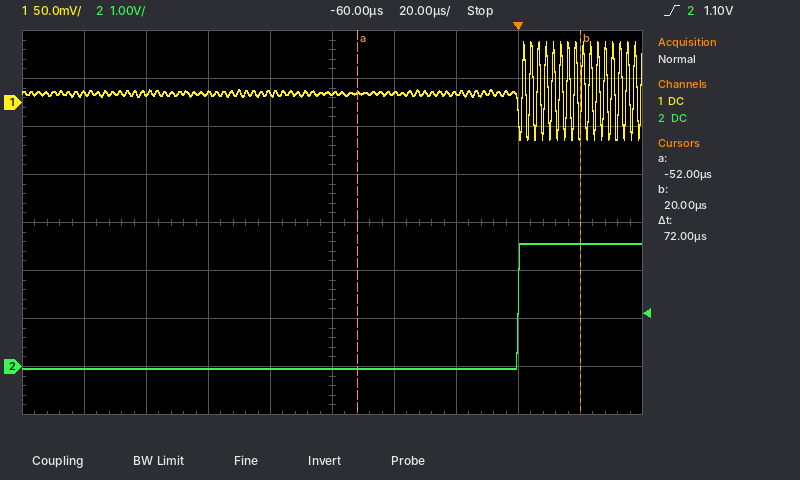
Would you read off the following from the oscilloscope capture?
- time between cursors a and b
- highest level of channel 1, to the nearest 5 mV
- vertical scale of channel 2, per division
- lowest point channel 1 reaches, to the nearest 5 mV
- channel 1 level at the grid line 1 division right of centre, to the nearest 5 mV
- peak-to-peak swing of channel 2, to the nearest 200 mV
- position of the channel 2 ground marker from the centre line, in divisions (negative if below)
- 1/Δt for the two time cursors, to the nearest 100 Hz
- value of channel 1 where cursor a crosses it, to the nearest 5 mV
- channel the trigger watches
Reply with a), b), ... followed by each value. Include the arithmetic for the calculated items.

a) 72 µs
b) 65 mV
c) 1 V
d) -40 mV
e) 10 mV
f) 2.6 V
g) -3.0 div
h) 1 / 72 µs ≈ 13.9 kHz
i) 10 mV
j) channel 2
